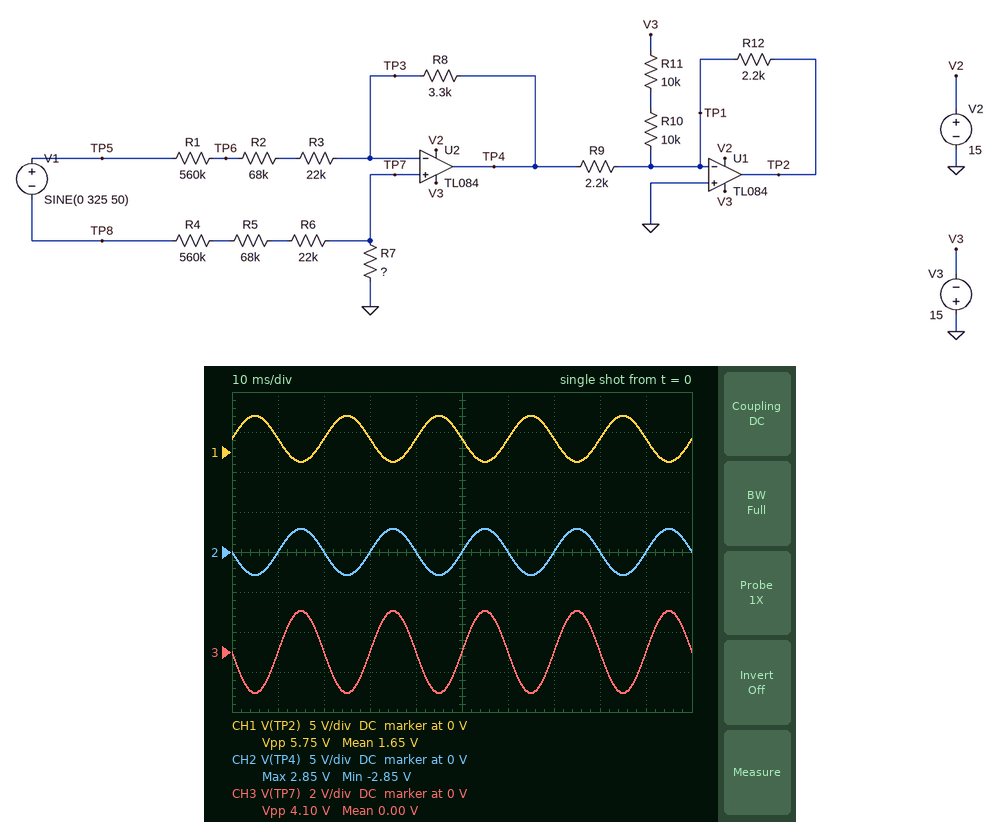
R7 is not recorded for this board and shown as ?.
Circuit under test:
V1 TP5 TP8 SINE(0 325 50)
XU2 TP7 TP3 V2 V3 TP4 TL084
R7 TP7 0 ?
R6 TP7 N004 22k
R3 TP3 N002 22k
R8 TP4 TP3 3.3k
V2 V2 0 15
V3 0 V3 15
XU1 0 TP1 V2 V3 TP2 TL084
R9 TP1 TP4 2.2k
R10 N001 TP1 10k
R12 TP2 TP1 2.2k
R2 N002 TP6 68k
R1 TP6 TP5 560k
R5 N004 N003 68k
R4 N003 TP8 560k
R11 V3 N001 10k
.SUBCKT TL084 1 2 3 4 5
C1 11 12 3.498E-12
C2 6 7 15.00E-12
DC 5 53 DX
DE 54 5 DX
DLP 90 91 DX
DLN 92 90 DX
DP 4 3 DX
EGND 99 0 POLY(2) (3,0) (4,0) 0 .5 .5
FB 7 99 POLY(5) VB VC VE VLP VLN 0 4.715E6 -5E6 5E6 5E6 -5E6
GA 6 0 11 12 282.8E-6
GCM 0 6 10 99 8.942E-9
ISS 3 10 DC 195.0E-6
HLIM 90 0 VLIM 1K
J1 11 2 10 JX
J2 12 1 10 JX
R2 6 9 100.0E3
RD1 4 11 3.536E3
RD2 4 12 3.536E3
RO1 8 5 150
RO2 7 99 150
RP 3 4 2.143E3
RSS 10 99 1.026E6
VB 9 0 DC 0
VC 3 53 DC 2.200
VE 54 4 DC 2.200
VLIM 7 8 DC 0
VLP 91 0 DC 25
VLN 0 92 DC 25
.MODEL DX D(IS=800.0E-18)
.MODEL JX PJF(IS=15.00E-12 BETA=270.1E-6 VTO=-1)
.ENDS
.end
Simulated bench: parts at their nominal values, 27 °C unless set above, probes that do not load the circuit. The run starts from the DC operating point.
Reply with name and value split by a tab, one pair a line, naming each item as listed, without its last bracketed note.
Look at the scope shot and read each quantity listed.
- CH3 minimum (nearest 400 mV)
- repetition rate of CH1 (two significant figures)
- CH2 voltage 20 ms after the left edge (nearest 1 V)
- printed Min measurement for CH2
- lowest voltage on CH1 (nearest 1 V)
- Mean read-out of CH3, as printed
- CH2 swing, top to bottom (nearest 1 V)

CH3 minimum	-2.0 V
repetition rate of CH1	50 Hz
CH2 voltage 20 ms after the left edge	0 V
printed Min measurement for CH2	-2.85 V
lowest voltage on CH1	-1 V
Mean read-out of CH3, as printed	0.00 V
CH2 swing, top to bottom	6 V
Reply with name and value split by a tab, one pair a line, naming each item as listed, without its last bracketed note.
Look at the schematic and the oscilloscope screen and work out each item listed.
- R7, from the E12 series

R7, from the E12 series	8.2 kΩ
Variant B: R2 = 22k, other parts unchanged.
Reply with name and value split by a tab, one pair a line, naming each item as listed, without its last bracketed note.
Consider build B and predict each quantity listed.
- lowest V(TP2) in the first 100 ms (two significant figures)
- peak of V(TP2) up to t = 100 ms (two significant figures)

lowest V(TP2) in the first 100 ms	-1.3 V
peak of V(TP2) up to t = 100 ms	4.6 V
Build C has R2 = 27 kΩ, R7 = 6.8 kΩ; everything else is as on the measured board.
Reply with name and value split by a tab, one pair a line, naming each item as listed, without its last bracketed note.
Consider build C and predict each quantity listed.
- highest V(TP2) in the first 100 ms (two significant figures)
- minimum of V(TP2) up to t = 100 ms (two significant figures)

highest V(TP2) in the first 100 ms	4.3 V
minimum of V(TP2) up to t = 100 ms	-960 mV
